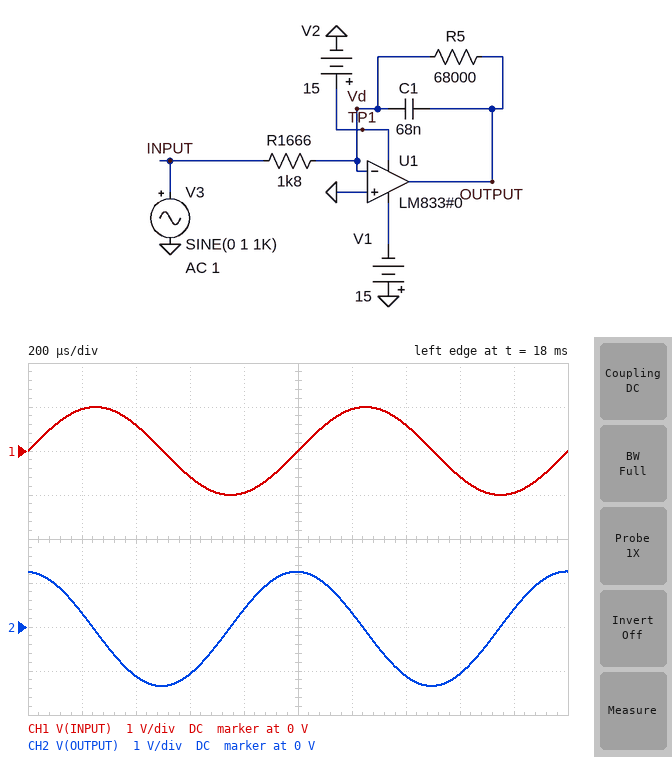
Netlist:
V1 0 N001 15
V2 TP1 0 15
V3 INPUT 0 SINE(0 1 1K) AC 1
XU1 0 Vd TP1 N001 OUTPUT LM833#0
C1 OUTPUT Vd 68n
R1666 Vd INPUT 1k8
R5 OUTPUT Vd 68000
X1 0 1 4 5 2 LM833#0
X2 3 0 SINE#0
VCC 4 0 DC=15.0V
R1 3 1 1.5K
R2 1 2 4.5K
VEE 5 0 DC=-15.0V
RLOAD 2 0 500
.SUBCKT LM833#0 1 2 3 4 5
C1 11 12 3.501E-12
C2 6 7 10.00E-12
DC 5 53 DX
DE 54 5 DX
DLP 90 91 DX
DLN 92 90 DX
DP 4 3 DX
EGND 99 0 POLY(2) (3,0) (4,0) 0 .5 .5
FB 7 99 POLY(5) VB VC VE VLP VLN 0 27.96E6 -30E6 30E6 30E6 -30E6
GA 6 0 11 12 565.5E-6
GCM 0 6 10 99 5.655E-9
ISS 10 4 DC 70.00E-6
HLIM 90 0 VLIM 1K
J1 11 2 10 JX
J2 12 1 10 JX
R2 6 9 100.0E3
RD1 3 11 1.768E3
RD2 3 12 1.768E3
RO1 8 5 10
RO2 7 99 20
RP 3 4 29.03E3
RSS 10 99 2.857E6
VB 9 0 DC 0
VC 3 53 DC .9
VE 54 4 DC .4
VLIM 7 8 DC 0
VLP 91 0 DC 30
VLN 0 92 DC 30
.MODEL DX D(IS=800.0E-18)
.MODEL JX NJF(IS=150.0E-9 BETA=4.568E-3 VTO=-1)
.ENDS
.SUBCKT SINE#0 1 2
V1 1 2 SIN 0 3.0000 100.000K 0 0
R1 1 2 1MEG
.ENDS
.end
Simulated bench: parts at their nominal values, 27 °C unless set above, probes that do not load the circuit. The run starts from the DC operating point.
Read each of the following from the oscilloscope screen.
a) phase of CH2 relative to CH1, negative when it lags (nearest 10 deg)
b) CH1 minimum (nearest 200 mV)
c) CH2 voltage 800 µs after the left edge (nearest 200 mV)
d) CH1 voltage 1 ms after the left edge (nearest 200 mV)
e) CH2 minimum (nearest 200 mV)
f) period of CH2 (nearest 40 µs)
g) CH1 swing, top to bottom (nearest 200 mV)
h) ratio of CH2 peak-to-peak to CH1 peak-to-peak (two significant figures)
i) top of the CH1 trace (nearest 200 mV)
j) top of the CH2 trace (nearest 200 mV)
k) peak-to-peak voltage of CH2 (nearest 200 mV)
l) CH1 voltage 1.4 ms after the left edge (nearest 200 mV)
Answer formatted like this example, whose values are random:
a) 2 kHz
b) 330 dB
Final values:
a) 90 deg
b) -1.0 V
c) 400 mV
d) 0 V
e) -1.4 V
f) 1.00 ms
g) 2.0 V
h) 1.3
i) 1.0 V
j) 1.2 V
k) 2.6 V
l) 600 mV
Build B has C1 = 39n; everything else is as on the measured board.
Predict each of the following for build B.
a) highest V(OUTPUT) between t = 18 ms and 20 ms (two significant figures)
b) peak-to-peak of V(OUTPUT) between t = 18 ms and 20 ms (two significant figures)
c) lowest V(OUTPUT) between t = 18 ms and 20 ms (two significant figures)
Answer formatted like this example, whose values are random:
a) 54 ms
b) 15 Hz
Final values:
a) 2.2 V
b) 4.5 V
c) -2.3 V
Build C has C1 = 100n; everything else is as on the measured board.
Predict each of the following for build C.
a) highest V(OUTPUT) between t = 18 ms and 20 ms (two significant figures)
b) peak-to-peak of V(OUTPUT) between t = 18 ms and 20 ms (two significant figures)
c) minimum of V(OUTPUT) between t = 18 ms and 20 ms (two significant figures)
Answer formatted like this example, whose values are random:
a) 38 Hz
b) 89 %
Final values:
a) 820 mV
b) 1.8 V
c) -960 mV
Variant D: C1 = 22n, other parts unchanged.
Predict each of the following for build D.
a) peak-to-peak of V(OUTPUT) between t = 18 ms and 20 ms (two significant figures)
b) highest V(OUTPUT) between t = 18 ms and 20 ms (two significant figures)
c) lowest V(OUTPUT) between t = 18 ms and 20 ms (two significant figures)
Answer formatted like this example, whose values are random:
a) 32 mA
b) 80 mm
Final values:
a) 8.0 V
b) 4.0 V
c) -4.0 V
